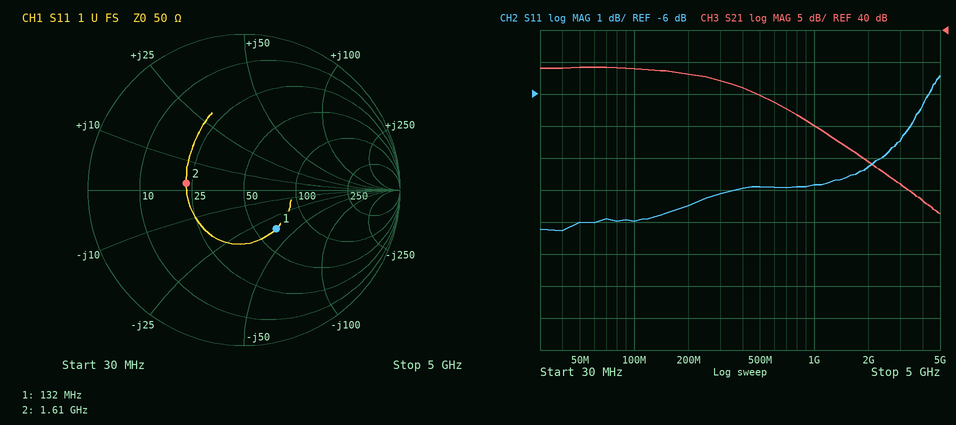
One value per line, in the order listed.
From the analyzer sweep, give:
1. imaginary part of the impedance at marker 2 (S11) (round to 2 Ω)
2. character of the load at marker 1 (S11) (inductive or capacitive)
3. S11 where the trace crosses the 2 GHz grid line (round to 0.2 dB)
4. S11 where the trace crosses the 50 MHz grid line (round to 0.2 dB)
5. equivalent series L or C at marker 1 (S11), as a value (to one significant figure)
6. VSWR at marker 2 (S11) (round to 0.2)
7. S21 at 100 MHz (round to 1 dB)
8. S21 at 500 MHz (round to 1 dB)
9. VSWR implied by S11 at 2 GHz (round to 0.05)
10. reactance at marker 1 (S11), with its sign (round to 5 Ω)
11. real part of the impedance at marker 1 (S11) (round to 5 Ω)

+2 Ω
capacitive
-8.2 dB
-10.0 dB
30 pF
2.2
34 dB
30 dB
2.25
-35 Ω
65 Ω
